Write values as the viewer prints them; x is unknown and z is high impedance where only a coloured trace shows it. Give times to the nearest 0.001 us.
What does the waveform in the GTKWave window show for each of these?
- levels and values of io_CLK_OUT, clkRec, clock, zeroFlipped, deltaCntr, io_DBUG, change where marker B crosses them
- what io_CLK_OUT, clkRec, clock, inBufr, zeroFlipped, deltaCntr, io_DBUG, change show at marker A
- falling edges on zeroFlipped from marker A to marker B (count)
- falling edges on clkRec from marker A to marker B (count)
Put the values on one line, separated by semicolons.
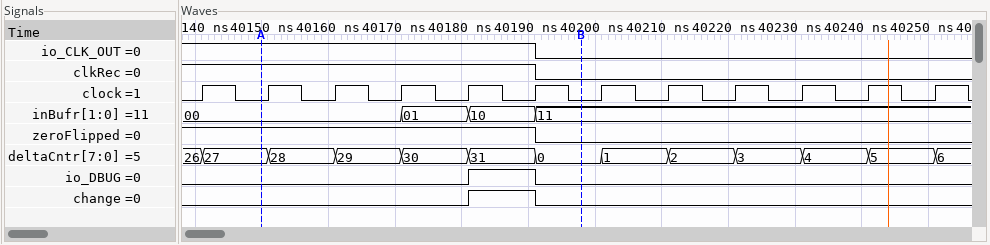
io_CLK_OUT=0, clkRec=0, clock=0, zeroFlipped=0, deltaCntr=0, io_DBUG=0, change=0; io_CLK_OUT=1, clkRec=1, clock=0, inBufr=00, zeroFlipped=1, deltaCntr=27, io_DBUG=0, change=0; 1; 1
